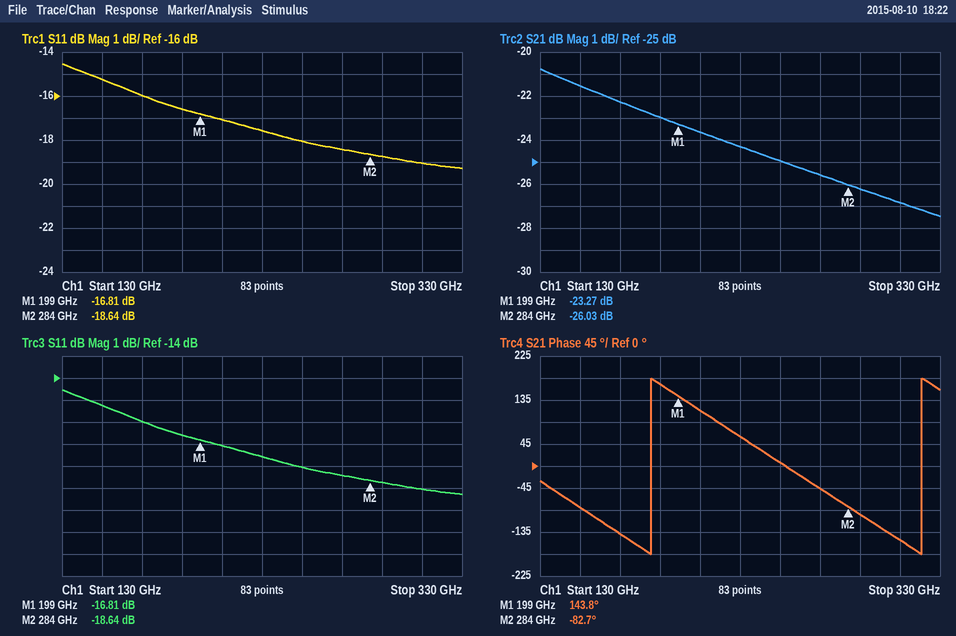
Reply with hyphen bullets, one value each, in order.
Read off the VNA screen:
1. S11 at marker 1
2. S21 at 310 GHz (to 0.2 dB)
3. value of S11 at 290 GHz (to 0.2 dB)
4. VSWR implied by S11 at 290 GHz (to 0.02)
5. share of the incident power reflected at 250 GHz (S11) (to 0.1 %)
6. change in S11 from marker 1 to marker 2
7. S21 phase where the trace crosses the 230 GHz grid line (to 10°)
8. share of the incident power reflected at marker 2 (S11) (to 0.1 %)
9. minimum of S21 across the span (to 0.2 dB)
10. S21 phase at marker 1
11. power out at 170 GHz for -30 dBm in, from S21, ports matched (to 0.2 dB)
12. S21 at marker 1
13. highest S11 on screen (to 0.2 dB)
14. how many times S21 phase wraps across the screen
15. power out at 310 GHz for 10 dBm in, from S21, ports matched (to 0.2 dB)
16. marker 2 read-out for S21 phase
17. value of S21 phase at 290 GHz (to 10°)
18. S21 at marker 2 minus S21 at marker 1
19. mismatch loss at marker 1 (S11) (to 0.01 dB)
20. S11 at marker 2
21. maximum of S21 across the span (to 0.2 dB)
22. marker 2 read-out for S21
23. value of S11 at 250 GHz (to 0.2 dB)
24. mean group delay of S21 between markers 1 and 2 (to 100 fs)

- -16.81 dB
- -26.8 dB
- -18.8 dB
- 1.26
- 1.6 %
- -1.83 dB
- 60°
- 1.4 %
- -27.4 dB
- 143.8°
- -52.2 dBm
- -23.27 dB
- -14.6 dB
- 2
- -16.8 dBm
- -82.7°
- -100°
- -2.76 dB
- 0.09 dB
- -18.64 dB
- -20.8 dB
- -26.03 dB
- -18.0 dB
- 7.4 ps
